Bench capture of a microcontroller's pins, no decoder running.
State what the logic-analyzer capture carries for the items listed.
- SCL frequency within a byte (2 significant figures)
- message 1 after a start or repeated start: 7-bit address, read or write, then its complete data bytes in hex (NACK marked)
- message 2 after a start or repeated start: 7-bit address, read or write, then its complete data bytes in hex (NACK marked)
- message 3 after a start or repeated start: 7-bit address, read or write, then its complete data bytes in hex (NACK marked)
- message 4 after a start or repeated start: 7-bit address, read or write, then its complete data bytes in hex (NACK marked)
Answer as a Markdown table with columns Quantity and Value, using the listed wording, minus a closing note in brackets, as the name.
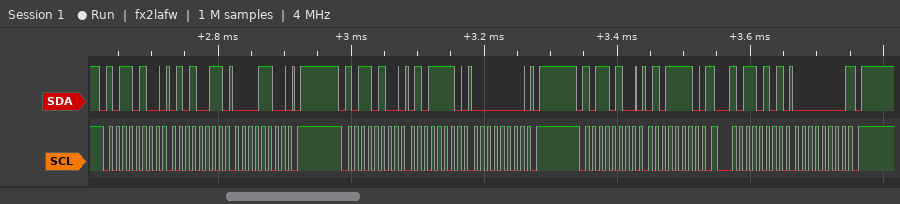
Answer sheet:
| Quantity | Value |
|---|---|
| SCL frequency within a byte | 100 kHz |
| message 1 after a start or repeated start: 7-bit address, read or write, then its complete data bytes in hex | 0x5A write: 53 0C |
| message 2 after a start or repeated start: 7-bit address, read or write, then its complete data bytes in hex | 0x5A write: 5E 00 |
| message 3 after a start or repeated start: 7-bit address, read or write, then its complete data bytes in hex | 0x5A write: 5E |
| message 4 after a start or repeated start: 7-bit address, read or write, then its complete data bytes in hex | 0x5A read: 00 NACK |
